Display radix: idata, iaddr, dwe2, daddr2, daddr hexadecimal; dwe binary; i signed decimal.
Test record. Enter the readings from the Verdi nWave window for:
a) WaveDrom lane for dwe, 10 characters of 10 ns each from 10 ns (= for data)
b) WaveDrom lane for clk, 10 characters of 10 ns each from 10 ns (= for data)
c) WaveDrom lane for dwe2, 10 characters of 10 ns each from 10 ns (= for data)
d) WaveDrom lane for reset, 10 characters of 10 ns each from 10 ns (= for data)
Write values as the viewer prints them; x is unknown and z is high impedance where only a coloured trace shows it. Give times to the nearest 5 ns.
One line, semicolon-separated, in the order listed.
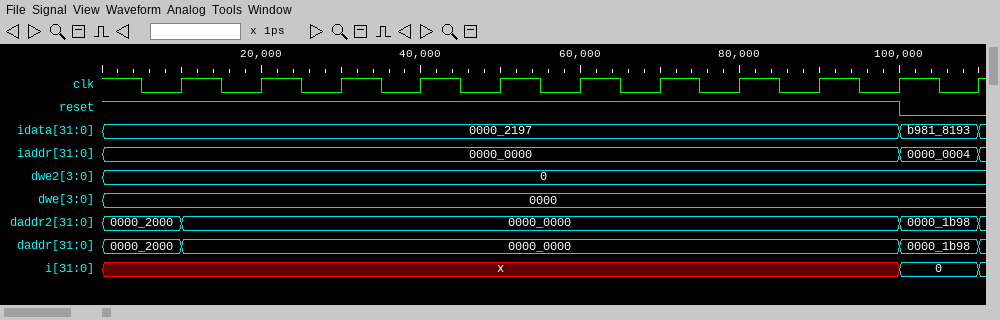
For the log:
{name: 'dwe', wave: '=.........', data: '0000'}; {name: 'clk', wave: 'p.........'}; {name: 'dwe2', wave: '=.........', data: '0'}; {name: 'reset', wave: '1........0'}
